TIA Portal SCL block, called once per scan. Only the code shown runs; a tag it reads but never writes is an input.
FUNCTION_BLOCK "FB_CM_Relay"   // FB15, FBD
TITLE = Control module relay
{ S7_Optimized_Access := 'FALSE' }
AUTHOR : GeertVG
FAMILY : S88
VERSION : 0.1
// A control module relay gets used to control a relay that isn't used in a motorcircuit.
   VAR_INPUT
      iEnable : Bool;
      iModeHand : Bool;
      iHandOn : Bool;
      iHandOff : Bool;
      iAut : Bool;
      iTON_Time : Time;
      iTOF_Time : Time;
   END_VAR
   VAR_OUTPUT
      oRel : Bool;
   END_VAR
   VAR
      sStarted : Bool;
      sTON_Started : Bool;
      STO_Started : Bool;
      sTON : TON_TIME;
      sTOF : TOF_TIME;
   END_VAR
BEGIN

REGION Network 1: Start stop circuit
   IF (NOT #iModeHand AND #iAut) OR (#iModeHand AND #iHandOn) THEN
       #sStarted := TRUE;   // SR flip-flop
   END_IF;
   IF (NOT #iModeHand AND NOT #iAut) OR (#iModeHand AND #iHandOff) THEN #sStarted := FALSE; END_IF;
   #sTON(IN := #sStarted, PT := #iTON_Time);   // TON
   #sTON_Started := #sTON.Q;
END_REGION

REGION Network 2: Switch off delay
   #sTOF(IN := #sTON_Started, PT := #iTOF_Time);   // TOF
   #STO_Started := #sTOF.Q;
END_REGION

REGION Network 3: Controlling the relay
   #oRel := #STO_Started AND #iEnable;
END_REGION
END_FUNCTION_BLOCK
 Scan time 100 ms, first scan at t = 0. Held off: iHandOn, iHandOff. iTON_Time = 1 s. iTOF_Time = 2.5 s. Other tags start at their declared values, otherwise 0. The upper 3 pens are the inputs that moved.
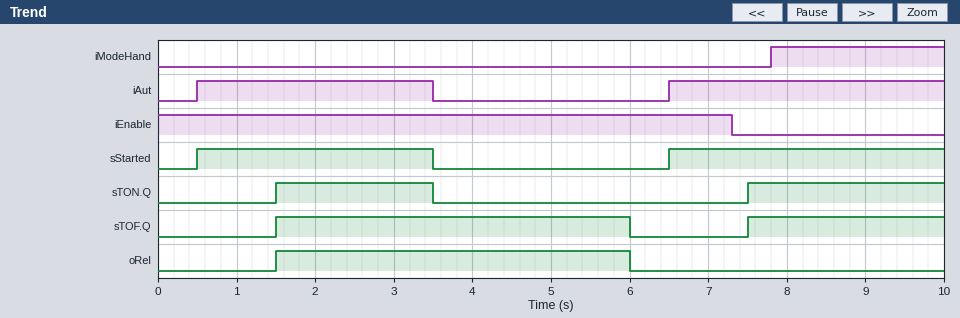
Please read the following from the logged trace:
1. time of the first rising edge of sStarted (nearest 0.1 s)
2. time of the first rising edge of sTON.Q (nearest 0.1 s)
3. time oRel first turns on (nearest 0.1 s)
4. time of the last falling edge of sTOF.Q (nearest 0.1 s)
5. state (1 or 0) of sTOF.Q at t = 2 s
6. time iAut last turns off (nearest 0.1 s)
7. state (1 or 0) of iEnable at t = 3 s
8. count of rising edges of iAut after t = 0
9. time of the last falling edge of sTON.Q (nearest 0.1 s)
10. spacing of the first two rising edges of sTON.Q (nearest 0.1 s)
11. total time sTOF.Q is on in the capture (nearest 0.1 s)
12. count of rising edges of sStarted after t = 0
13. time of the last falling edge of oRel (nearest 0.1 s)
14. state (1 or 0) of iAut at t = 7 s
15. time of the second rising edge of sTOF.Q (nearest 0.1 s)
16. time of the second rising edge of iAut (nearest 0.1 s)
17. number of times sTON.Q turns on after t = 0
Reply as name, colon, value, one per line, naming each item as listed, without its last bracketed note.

time of the first rising edge of sStarted: 0.5 s
time of the first rising edge of sTON.Q: 1.5 s
time oRel first turns on: 1.5 s
time of the last falling edge of sTOF.Q: 6.0 s
state (1 or 0) of sTOF.Q at t = 2 s: 1
time iAut last turns off: 3.5 s
state (1 or 0) of iEnable at t = 3 s: 1
count of rising edges of iAut after t = 0: 2
time of the last falling edge of sTON.Q: 3.5 s
spacing of the first two rising edges of sTON.Q: 6.0 s
total time sTOF.Q is on in the capture: 7.0 s
count of rising edges of sStarted after t = 0: 2
time of the last falling edge of oRel: 6.0 s
state (1 or 0) of iAut at t = 7 s: 1
time of the second rising edge of sTOF.Q: 7.5 s
time of the second rising edge of iAut: 6.5 s
number of times sTON.Q turns on after t = 0: 2
